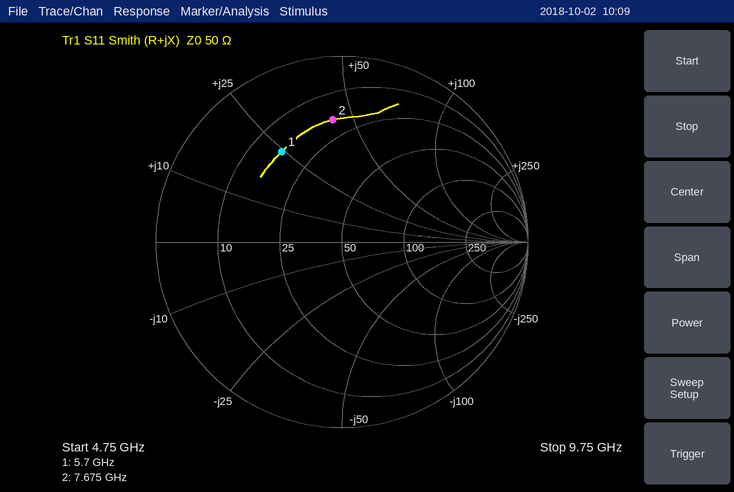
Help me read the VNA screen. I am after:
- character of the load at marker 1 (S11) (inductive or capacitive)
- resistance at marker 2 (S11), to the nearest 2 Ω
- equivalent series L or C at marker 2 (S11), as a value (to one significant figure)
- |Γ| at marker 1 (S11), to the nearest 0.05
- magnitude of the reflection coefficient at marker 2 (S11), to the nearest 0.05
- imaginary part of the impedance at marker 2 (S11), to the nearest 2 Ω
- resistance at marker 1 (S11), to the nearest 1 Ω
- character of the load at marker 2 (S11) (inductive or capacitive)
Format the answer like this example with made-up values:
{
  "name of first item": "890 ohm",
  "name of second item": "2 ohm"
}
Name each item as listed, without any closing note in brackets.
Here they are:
{
  "character of the load at marker 1 (S11)": "inductive",
  "resistance at marker 2 (S11), to the nearest 2 Ω": "18 Ω",
  "equivalent series L or C at marker 2 (S11), as a value": "900 pH",
  "|Γ| at marker 1 (S11), to the nearest 0.05": "0.60",
  "magnitude of the reflection coefficient at marker 2 (S11), to the nearest 0.05": "0.65",
  "imaginary part of the impedance at marker 2 (S11), to the nearest 2 Ω": "+42 Ω",
  "resistance at marker 1 (S11), to the nearest 1 Ω": "17 Ω",
  "character of the load at marker 2 (S11)": "inductive"
}
